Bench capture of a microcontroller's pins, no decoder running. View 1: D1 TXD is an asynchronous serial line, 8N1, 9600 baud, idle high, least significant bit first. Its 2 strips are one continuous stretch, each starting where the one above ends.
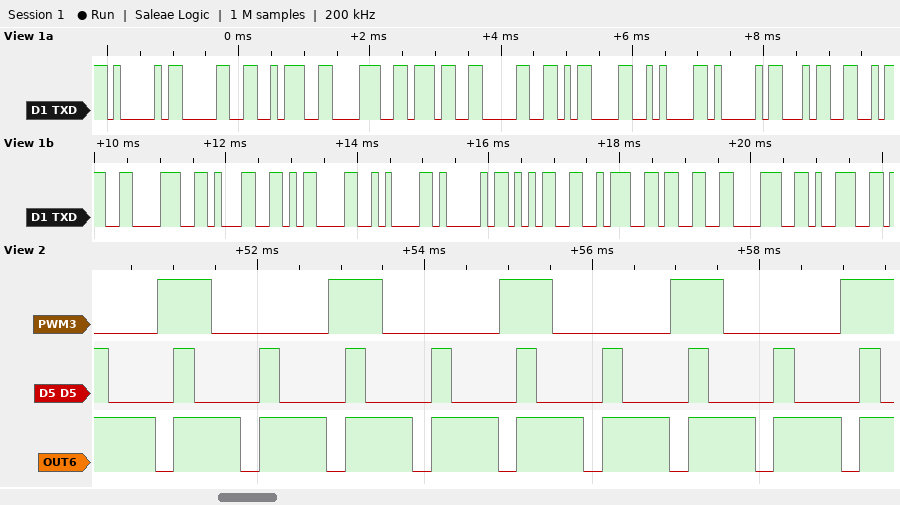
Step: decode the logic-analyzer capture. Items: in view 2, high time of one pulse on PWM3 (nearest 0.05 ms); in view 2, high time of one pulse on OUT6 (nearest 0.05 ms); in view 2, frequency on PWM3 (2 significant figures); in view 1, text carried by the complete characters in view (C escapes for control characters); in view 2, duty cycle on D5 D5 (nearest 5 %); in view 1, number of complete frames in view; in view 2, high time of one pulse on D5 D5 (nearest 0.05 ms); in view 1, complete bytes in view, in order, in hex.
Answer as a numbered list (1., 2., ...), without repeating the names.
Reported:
1. 0.65 ms
2. 0.80 ms
3. 490 Hz
4. "A0:870\r\nA4:81\r\nA5:389"
5. 25 %
6. 21
7. 0.25 ms
8. 0x41 0x30 0x3A 0x38 0x37 0x30 0x0D 0x0A 0x41 0x34 0x3A 0x38 0x31 0x0D 0x0A 0x41 0x35 0x3A 0x33 0x38 0x39
